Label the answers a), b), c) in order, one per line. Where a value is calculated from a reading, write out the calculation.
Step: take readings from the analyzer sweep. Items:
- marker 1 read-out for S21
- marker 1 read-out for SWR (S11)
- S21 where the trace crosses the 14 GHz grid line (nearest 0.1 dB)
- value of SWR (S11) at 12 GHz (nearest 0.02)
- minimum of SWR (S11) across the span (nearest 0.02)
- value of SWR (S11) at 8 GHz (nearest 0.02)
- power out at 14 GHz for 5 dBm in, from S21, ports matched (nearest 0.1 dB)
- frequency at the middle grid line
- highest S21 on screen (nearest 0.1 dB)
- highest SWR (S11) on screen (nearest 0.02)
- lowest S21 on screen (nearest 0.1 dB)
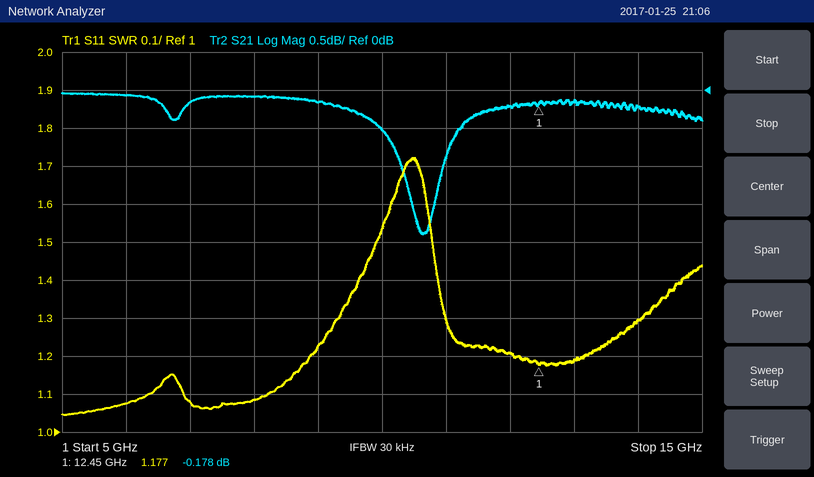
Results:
a) -0.178 dB
b) 1.177
c) -0.2 dB
d) 1.20
e) 1.04
f) 1.08
g) 5 dBm + (-0.2 dB) = 4.8 dBm
h) 10 GHz
i) 0.0 dB
j) 1.72
k) -1.9 dB
